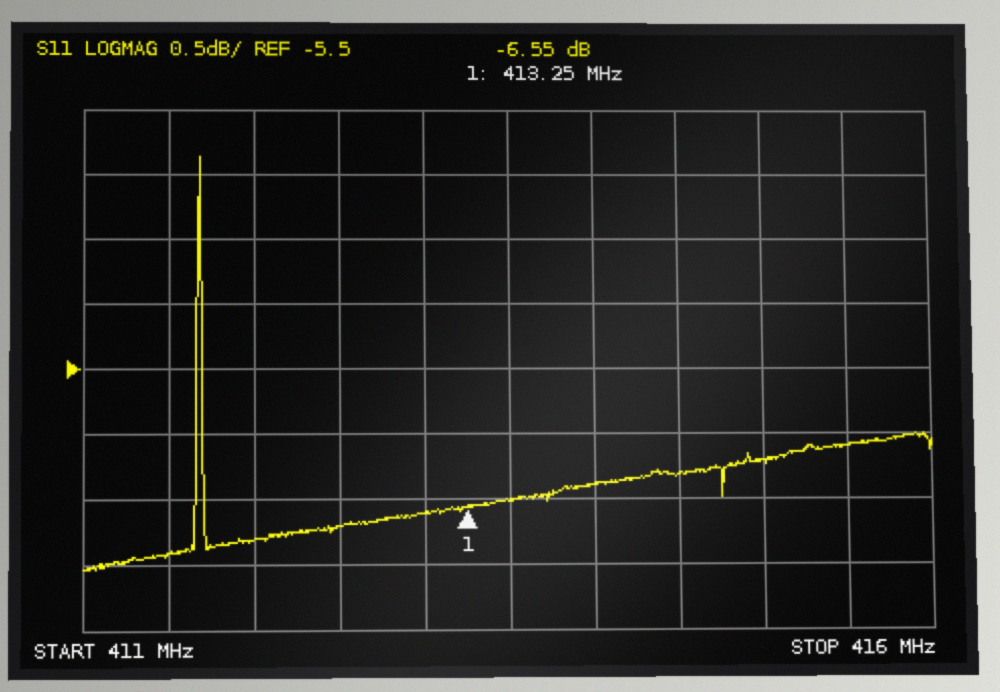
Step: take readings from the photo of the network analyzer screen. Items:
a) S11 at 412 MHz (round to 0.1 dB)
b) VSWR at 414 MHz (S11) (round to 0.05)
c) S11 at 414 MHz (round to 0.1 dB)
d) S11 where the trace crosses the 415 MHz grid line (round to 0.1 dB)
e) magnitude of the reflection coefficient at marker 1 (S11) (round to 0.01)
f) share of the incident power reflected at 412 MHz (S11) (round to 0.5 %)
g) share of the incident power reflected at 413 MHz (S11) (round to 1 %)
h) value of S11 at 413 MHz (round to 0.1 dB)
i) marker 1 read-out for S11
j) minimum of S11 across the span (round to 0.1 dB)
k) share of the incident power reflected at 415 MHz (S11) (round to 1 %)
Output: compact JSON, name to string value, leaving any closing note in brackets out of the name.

{"S11 at 412 MHz": "-6.8 dB", "VSWR at 414 MHz (S11)": "2.85", "S11 at 414 MHz": "-6.4 dB", "S11 where the trace crosses the 415 MHz grid line": "-6.2 dB", "magnitude of the reflection coefficient at marker 1 (S11)": "0.47", "share of the incident power reflected at 412 MHz (S11)": "21.0 %", "share of the incident power reflected at 413 MHz (S11)": "22 %", "value of S11 at 413 MHz": "-6.6 dB", "marker 1 read-out for S11": "-6.55 dB", "minimum of S11 across the span": "-7.0 dB", "share of the incident power reflected at 415 MHz (S11)": "24 %"}
